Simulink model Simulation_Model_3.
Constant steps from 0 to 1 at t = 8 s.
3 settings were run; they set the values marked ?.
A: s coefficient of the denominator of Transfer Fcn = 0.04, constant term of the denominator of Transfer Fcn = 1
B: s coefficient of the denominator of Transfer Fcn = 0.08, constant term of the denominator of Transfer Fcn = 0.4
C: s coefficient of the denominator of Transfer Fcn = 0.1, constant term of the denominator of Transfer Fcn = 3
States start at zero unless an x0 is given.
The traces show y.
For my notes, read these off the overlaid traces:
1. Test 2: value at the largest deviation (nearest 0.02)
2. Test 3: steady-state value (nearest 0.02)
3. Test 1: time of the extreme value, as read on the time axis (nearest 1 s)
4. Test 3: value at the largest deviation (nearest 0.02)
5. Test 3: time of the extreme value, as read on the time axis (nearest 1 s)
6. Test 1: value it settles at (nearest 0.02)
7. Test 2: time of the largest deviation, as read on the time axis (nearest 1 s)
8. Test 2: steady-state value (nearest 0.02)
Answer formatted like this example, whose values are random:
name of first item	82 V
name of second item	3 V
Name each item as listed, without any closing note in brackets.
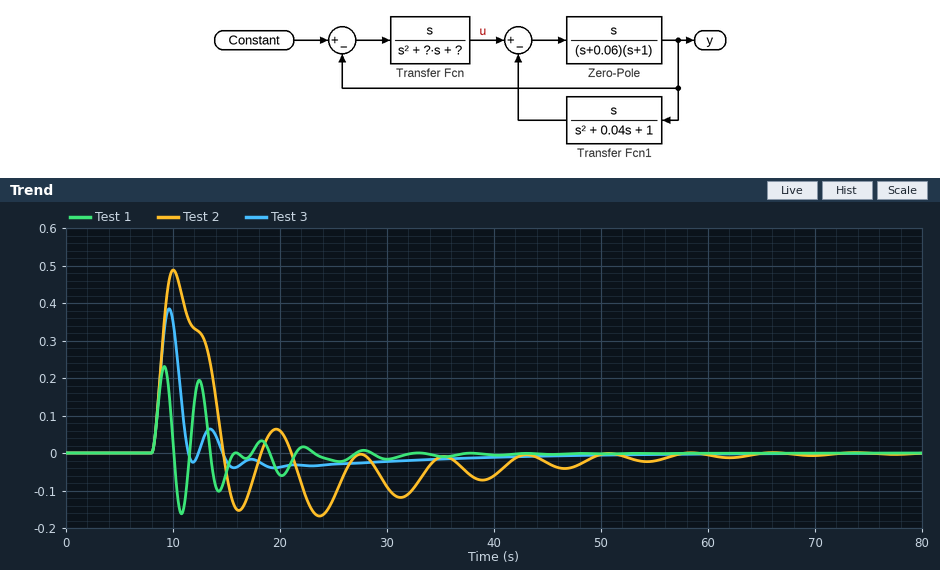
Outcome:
Test 2: value at the largest deviation	0.48
Test 3: steady-state value	0.00
Test 1: time of the extreme value, as read on the time axis	9 s
Test 3: value at the largest deviation	0.38
Test 3: time of the extreme value, as read on the time axis	10 s
Test 1: value it settles at	0.00
Test 2: time of the largest deviation, as read on the time axis	10 s
Test 2: steady-state value	0.00
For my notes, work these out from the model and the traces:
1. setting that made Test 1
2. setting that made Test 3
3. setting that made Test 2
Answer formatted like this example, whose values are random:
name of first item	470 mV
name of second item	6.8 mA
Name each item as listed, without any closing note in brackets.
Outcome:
setting that made Test 1	C
setting that made Test 3	A
setting that made Test 2	B
